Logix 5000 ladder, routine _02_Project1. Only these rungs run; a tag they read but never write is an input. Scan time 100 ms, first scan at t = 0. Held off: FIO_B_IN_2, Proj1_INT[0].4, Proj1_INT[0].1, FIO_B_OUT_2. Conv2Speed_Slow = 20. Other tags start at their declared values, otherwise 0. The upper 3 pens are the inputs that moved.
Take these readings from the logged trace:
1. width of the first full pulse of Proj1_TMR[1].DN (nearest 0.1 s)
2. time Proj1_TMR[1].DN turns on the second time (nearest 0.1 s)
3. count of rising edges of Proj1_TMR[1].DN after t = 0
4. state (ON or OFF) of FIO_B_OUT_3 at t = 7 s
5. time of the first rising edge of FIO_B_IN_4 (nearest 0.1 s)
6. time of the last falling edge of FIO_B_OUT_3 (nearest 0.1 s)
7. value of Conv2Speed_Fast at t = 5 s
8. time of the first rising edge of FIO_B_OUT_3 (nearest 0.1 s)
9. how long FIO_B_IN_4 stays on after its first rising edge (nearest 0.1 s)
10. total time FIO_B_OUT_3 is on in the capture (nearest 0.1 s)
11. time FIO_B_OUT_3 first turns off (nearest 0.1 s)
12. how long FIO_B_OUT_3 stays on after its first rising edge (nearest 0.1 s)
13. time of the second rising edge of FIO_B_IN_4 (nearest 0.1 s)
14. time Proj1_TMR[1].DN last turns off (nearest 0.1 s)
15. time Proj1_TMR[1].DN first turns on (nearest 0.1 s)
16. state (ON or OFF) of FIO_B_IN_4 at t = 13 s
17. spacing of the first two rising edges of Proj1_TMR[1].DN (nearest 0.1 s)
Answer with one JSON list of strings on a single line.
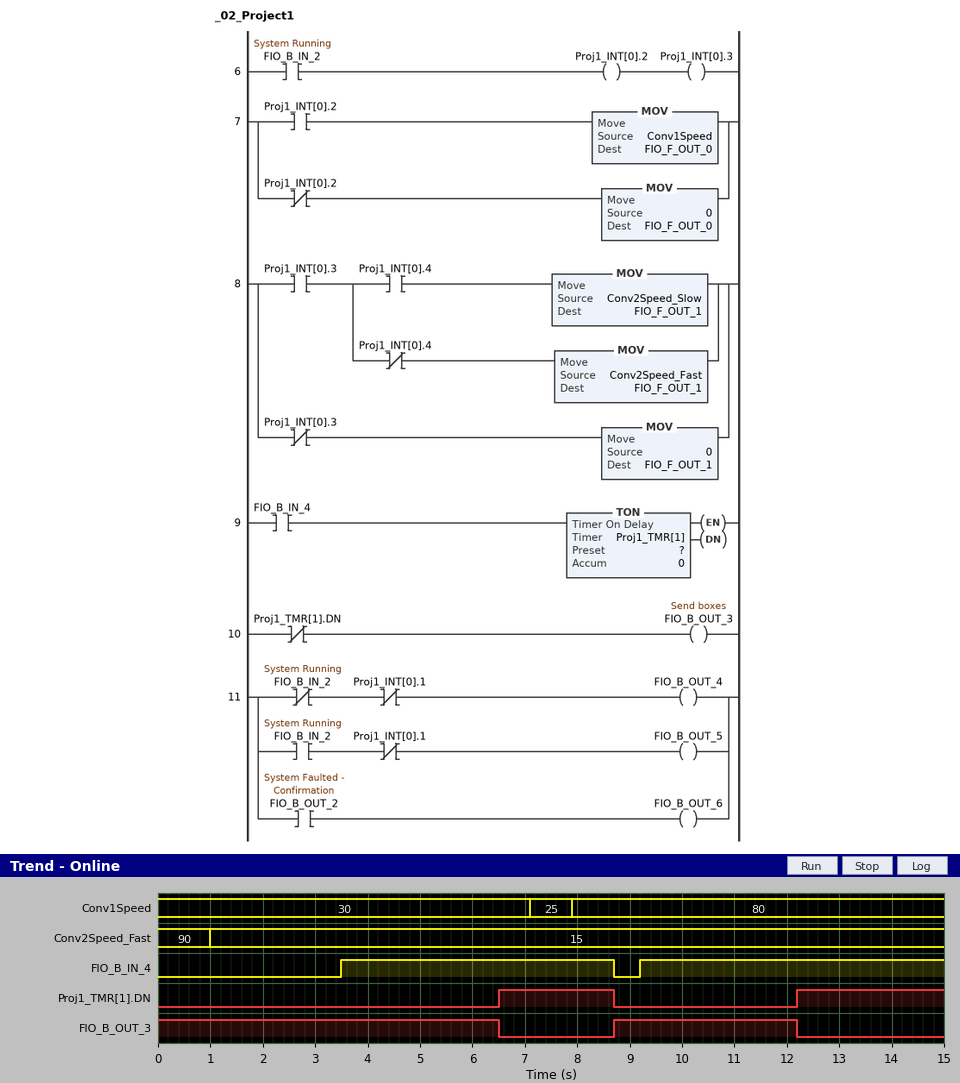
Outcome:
["2.2 s", "12.2 s", "2", "OFF", "3.5 s", "12.2 s", "15", "8.7 s", "5.2 s", "10.0 s", "6.5 s", "3.5 s", "9.2 s", "8.7 s", "6.5 s", "ON", "5.7 s"]
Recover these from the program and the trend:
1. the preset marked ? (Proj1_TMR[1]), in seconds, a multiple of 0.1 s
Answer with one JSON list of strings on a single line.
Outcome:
["3.0 s"]
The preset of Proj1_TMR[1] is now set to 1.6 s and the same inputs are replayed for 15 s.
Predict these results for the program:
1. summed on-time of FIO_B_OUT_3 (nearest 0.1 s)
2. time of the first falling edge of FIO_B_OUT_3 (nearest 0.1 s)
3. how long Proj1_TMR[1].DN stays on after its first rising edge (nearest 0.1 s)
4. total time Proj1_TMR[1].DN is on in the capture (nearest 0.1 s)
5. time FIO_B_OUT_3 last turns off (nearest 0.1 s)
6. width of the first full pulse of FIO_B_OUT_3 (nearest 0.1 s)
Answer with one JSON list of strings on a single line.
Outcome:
["7.2 s", "5.1 s", "3.6 s", "7.8 s", "10.8 s", "2.1 s"]
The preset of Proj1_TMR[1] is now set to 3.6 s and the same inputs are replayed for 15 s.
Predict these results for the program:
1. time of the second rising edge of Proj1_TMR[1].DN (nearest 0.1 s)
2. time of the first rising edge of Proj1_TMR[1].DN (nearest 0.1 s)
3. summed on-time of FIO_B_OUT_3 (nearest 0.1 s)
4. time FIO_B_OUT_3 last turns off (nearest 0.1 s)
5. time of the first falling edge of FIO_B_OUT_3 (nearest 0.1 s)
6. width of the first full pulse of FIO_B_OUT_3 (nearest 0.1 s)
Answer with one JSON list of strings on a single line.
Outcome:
["12.8 s", "7.1 s", "11.2 s", "12.8 s", "7.1 s", "4.1 s"]
